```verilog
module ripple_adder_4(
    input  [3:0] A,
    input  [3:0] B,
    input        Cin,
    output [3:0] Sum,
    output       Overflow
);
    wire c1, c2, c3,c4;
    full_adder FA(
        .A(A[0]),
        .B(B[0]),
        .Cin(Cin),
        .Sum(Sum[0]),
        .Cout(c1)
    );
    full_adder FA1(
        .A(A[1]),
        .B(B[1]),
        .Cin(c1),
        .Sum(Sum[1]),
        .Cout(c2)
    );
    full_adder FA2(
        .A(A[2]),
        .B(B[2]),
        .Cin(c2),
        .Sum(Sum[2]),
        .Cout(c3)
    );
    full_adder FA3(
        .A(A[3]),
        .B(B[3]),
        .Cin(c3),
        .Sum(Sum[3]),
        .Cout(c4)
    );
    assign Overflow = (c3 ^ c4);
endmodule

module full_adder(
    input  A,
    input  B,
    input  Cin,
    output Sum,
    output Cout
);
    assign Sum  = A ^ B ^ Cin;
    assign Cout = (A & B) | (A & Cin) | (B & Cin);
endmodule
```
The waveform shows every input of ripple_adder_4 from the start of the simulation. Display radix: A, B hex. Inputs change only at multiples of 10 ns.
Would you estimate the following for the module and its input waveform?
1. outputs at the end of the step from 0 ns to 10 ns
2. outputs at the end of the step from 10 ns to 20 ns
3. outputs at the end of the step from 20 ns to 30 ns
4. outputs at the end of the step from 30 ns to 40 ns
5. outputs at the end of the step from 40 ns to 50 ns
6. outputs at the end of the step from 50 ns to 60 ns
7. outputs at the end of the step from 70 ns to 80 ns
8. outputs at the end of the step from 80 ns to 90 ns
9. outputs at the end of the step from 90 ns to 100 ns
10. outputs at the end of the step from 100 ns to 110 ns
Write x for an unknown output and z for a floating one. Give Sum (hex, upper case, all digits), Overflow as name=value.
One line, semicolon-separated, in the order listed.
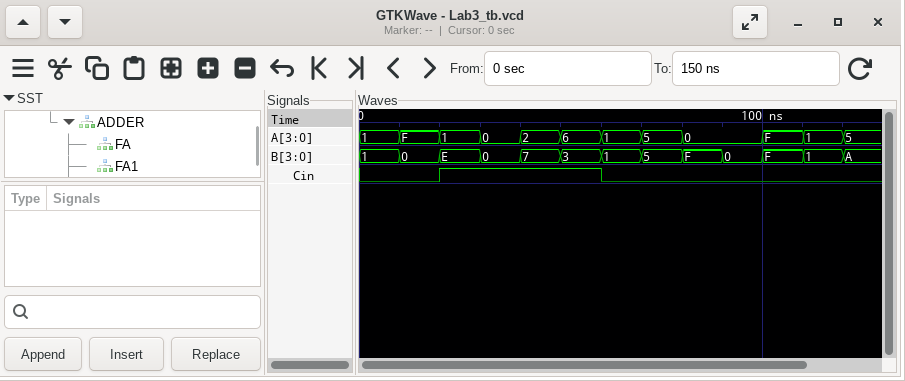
Sum=2, Overflow=0; Sum=F, Overflow=0; Sum=0, Overflow=0; Sum=1, Overflow=0; Sum=A, Overflow=1; Sum=A, Overflow=1; Sum=A, Overflow=1; Sum=F, Overflow=0; Sum=0, Overflow=0; Sum=E, Overflow=0
